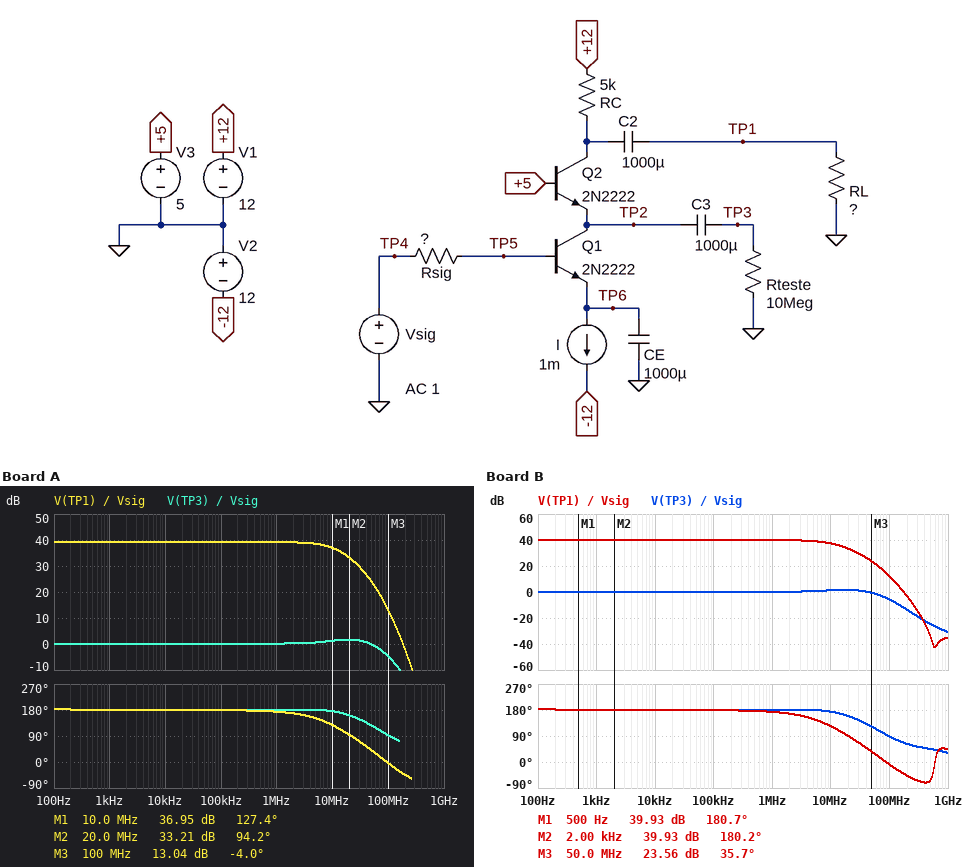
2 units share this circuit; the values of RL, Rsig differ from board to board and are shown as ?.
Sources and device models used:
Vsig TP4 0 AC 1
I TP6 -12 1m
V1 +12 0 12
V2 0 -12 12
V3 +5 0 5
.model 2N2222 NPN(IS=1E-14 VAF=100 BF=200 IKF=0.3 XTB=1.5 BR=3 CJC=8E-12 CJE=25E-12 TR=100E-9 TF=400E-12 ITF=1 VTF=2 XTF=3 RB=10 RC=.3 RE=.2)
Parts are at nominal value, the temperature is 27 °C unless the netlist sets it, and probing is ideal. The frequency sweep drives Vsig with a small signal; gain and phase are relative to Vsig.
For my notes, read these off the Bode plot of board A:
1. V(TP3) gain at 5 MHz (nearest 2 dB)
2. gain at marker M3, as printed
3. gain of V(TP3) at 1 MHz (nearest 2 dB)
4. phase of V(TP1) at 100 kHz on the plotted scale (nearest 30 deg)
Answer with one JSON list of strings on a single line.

["0 dB", "13.04 dB", "0 dB", "180 deg"]
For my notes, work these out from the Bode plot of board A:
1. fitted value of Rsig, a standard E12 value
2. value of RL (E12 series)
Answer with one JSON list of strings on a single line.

["27 Ω", "4.7 kΩ"]
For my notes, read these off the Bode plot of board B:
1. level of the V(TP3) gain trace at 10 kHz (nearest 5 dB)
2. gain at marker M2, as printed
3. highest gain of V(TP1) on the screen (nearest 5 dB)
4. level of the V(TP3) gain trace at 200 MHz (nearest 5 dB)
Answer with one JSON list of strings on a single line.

["0 dB", "39.93 dB", "40 dB", "-15 dB"]
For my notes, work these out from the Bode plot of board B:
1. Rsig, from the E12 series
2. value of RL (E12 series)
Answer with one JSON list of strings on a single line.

["33 Ω", "5.6 kΩ"]
